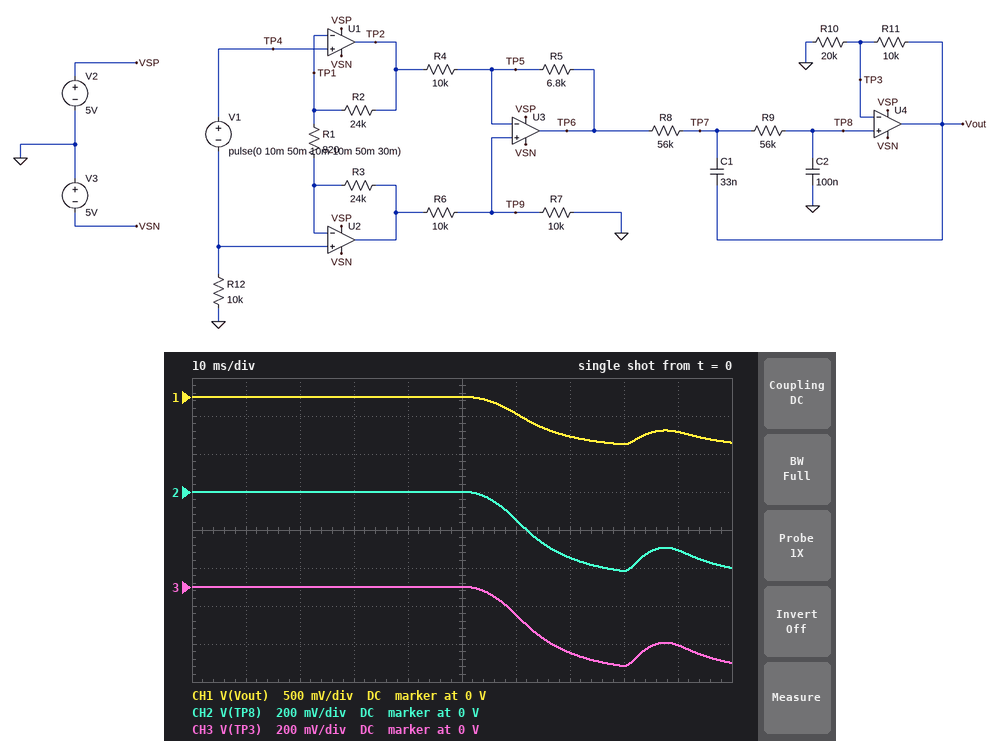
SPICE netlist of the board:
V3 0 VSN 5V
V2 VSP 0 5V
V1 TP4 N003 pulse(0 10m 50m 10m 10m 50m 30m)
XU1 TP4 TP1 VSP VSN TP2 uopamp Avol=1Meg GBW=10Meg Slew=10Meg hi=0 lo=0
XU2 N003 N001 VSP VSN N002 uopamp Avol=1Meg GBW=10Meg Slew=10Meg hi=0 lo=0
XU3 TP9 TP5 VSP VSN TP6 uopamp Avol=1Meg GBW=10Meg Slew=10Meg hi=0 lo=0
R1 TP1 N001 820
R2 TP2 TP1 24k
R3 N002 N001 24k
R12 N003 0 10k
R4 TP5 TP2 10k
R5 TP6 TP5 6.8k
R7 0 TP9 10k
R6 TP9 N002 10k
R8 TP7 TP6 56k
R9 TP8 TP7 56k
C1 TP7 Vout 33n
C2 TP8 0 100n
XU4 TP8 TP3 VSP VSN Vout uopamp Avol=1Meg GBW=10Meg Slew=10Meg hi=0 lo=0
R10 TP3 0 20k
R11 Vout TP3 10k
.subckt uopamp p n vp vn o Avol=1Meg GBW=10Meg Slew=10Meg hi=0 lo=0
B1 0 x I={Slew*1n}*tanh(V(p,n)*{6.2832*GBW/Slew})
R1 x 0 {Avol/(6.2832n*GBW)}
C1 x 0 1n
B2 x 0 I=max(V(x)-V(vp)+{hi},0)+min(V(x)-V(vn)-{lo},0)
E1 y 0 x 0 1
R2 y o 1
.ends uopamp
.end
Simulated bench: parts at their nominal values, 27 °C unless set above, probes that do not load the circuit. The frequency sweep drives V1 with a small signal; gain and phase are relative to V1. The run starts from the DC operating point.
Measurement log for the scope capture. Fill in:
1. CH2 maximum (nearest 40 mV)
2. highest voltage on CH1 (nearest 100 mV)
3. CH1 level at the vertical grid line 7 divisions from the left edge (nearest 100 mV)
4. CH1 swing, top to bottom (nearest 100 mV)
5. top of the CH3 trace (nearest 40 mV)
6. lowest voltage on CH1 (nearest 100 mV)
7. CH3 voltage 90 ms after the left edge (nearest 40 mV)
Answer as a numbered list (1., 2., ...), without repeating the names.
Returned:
1. 0 V
2. 0 V
3. -500 mV
4. 600 mV
5. 0 V
6. -600 mV
7. -320 mV
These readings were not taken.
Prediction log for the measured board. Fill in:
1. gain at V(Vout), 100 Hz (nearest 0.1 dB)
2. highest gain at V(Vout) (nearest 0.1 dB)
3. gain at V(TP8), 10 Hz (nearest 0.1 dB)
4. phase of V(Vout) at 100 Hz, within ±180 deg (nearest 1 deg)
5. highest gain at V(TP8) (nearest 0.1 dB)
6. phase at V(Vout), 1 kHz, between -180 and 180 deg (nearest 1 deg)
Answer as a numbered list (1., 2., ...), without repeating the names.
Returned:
1. 19.5 dB
2. 36.6 dB
3. 31.8 dB
4. 64 deg
5. 33.1 dB
6. 9 deg
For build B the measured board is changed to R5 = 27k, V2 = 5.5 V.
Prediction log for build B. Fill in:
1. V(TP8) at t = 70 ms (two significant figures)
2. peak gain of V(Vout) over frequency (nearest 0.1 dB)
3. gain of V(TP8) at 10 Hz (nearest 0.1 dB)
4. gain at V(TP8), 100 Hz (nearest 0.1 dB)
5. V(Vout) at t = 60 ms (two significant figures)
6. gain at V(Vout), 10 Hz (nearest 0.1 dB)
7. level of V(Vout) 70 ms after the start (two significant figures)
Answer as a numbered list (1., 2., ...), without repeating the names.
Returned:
1. -1.0 V
2. 46.2 dB
3. 41.4 dB
4. 25.6 dB
5. -660 mV
6. 44.9 dB
7. -1.6 V
